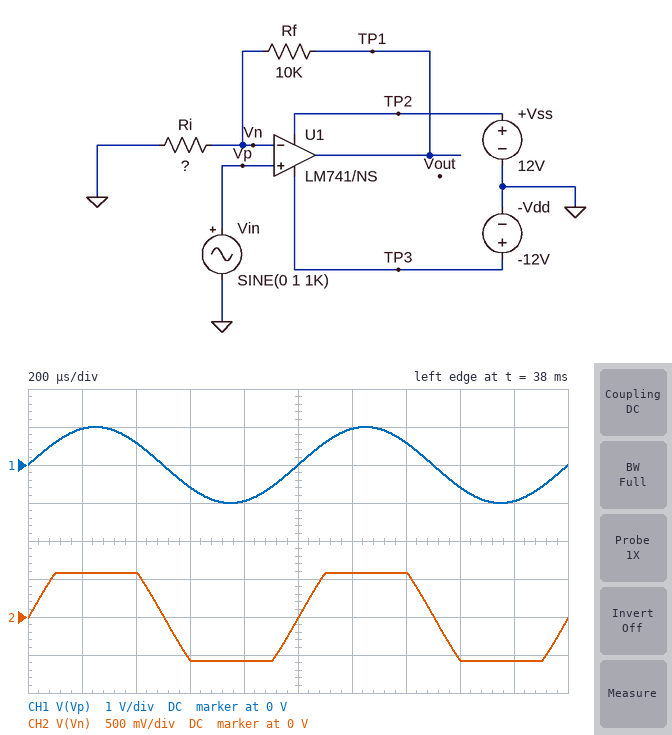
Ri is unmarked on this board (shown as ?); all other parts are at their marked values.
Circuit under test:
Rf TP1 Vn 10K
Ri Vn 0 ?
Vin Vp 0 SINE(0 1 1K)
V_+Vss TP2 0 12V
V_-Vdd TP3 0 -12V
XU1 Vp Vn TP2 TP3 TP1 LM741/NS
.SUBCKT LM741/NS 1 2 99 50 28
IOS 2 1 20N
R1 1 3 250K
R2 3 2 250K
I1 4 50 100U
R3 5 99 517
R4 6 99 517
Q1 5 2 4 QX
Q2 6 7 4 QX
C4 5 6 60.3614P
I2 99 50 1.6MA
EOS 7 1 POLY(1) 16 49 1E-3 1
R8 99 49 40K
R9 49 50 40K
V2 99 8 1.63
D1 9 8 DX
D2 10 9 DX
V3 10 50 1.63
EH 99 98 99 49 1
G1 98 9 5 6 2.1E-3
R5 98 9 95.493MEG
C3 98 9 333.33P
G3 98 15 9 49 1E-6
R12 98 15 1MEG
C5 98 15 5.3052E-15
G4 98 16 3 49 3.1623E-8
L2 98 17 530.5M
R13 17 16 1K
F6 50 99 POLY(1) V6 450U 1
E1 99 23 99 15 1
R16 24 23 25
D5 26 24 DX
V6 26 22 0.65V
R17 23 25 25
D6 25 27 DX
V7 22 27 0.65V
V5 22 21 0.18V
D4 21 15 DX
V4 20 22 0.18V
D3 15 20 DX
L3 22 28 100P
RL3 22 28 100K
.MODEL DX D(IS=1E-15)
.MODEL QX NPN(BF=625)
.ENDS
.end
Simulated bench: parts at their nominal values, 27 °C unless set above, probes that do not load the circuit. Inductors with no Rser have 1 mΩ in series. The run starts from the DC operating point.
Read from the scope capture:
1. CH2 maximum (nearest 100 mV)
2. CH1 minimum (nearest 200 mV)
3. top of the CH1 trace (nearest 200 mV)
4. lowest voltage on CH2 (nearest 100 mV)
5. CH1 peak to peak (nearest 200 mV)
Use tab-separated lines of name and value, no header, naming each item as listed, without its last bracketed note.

CH2 maximum	600 mV
CH1 minimum	-1.0 V
top of the CH1 trace	1.0 V
lowest voltage on CH2	-600 mV
CH1 peak to peak	2.0 V
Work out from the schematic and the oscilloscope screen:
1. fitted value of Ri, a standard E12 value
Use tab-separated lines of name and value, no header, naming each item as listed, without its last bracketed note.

fitted value of Ri, a standard E12 value	560 Ω
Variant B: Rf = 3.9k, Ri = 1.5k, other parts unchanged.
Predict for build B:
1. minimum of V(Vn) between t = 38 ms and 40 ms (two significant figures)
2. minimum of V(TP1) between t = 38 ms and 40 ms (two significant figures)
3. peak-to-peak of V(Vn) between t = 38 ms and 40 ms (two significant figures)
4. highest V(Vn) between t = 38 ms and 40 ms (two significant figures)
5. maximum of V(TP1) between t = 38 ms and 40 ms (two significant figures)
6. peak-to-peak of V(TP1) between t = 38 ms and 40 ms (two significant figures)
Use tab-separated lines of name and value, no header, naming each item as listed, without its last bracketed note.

minimum of V(Vn) between t = 38 ms and 40 ms	-1.0 V
minimum of V(TP1) between t = 38 ms and 40 ms	-3.6 V
peak-to-peak of V(Vn) between t = 38 ms and 40 ms	2.0 V
highest V(Vn) between t = 38 ms and 40 ms	1.0 V
maximum of V(TP1) between t = 38 ms and 40 ms	3.6 V
peak-to-peak of V(TP1) between t = 38 ms and 40 ms	7.2 V
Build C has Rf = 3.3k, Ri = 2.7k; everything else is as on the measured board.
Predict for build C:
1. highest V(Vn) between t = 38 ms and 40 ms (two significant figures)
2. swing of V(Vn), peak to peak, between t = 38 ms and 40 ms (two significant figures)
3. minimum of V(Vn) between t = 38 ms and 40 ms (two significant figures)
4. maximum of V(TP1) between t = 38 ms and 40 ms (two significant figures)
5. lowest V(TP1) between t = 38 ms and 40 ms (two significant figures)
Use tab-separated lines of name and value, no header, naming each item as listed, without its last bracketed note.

highest V(Vn) between t = 38 ms and 40 ms	1.0 V
swing of V(Vn), peak to peak, between t = 38 ms and 40 ms	2.0 V
minimum of V(Vn) between t = 38 ms and 40 ms	-1.0 V
maximum of V(TP1) between t = 38 ms and 40 ms	2.2 V
lowest V(TP1) between t = 38 ms and 40 ms	-2.2 V
